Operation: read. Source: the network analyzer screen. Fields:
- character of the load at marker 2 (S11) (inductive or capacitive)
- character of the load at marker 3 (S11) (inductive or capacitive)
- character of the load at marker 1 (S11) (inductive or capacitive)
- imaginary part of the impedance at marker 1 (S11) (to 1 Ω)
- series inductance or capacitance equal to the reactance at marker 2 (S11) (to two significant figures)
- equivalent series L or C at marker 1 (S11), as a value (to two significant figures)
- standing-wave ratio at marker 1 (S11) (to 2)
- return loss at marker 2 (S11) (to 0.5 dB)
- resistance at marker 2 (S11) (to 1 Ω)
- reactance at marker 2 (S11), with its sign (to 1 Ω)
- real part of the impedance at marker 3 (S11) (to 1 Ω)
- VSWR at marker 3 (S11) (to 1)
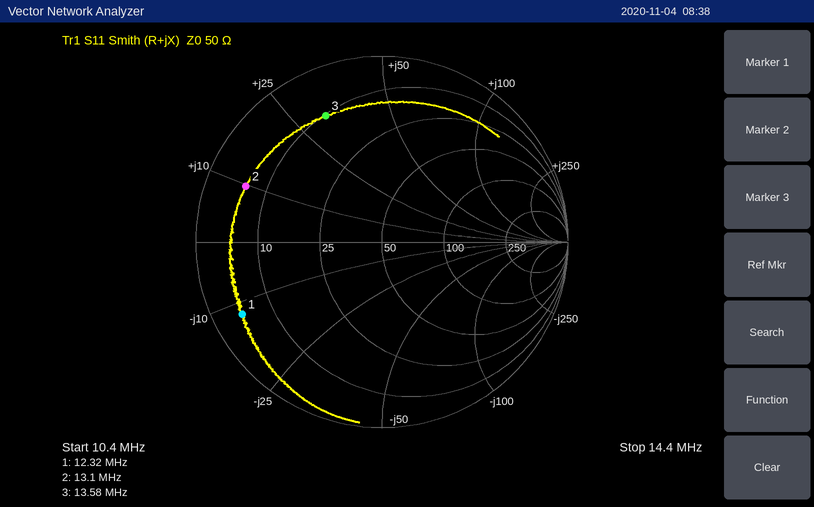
inductive
inductive
capacitive
-12 Ω
120 nH
1.1 nF
12
2.0 dB
6 Ω
+10 Ω
10 Ω
7
